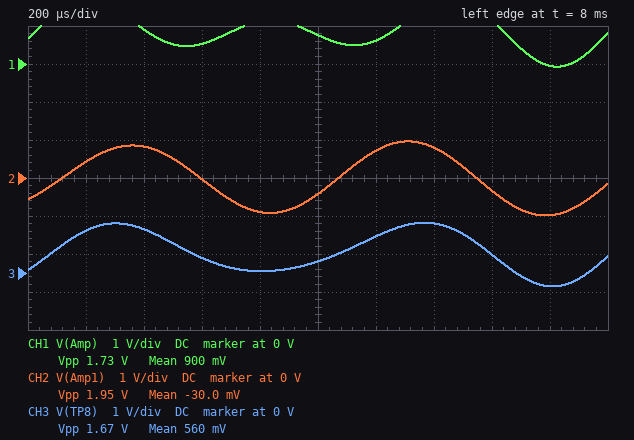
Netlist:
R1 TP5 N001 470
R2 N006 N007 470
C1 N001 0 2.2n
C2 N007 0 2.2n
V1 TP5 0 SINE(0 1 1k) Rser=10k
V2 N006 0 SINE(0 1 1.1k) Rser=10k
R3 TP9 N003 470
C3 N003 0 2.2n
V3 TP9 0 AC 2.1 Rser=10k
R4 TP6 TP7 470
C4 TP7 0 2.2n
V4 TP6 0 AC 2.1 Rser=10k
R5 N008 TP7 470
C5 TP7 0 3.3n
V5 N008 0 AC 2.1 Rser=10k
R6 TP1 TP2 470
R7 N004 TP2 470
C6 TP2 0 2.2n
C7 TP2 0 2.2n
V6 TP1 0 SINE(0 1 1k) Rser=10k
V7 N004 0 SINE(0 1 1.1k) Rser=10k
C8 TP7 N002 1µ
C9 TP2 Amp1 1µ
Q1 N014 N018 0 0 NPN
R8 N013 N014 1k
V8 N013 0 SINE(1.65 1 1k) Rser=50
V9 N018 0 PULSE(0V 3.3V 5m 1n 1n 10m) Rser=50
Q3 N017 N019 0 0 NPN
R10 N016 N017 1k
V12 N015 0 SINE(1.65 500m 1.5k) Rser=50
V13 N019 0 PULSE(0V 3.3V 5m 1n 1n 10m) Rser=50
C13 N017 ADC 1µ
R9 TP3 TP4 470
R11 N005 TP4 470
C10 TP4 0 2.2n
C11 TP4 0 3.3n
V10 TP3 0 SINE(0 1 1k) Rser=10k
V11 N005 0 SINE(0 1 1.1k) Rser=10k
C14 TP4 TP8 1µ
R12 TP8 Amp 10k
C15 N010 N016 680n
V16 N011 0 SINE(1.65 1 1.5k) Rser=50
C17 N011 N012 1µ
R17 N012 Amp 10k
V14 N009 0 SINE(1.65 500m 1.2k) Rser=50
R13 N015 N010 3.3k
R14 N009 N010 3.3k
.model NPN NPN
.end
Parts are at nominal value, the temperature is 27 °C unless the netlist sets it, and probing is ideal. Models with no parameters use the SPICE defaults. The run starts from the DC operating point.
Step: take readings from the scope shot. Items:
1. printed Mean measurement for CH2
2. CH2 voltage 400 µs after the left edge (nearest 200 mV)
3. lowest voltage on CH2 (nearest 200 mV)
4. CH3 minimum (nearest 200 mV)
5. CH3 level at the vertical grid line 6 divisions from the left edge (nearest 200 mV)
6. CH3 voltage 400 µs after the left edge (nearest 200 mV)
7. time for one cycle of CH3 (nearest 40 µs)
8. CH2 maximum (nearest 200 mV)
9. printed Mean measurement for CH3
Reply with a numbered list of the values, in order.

1. -30.0 mV
2. 800 mV
3. -1.0 V
4. -400 mV
5. 1.0 V
6. 1.2 V
7. 1.00 ms
8. 1.0 V
9. 560 mV
